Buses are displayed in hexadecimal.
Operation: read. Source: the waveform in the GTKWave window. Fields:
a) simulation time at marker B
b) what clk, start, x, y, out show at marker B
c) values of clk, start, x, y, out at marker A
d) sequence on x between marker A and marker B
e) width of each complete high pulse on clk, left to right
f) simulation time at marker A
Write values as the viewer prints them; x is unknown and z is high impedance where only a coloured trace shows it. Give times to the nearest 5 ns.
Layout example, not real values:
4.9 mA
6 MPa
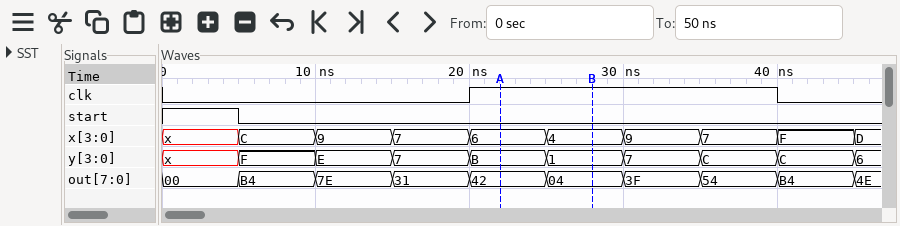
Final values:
30 ns
clk=1, start=0, x=4, y=1, out=04
clk=1, start=0, x=6, y=B, out=42
6, 4
20 ns
20 ns
